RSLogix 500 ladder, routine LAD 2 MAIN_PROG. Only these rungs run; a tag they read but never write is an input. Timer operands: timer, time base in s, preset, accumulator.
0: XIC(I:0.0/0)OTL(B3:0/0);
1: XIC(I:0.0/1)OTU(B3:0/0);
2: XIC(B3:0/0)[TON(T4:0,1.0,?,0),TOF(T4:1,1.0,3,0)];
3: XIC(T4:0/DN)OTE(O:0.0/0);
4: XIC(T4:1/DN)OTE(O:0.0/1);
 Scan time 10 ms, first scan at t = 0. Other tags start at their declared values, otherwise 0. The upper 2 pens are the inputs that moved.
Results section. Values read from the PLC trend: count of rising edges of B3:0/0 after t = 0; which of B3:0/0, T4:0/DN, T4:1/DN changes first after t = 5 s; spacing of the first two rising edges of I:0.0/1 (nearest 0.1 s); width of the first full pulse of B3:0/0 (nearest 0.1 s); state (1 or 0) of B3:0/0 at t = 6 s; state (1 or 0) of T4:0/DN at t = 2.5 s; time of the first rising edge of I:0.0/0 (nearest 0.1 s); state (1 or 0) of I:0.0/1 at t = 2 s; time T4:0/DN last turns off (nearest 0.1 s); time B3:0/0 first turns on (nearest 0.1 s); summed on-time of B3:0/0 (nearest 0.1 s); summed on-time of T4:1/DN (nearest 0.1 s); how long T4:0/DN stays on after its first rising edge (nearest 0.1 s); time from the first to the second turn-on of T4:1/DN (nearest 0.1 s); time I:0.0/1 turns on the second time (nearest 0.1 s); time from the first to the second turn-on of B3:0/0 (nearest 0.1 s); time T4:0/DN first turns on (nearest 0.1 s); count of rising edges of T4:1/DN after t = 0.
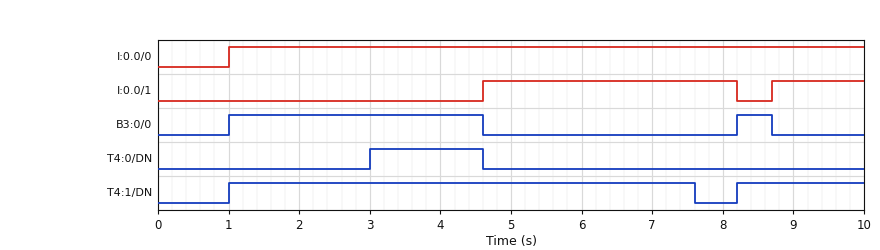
2
T4:1/DN
4.1 s
3.6 s
0
0
1.0 s
0
4.6 s
1.0 s
4.1 s
8.4 s
1.6 s
7.2 s
8.7 s
7.2 s
3.0 s
2
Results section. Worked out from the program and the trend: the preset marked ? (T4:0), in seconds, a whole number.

2 s
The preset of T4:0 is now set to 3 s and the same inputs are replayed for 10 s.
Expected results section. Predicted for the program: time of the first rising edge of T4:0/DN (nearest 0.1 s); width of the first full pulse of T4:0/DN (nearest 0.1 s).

4.0 s
0.6 s
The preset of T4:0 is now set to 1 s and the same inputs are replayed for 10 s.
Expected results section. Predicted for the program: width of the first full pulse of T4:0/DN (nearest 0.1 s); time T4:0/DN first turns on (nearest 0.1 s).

2.6 s
2.0 s
